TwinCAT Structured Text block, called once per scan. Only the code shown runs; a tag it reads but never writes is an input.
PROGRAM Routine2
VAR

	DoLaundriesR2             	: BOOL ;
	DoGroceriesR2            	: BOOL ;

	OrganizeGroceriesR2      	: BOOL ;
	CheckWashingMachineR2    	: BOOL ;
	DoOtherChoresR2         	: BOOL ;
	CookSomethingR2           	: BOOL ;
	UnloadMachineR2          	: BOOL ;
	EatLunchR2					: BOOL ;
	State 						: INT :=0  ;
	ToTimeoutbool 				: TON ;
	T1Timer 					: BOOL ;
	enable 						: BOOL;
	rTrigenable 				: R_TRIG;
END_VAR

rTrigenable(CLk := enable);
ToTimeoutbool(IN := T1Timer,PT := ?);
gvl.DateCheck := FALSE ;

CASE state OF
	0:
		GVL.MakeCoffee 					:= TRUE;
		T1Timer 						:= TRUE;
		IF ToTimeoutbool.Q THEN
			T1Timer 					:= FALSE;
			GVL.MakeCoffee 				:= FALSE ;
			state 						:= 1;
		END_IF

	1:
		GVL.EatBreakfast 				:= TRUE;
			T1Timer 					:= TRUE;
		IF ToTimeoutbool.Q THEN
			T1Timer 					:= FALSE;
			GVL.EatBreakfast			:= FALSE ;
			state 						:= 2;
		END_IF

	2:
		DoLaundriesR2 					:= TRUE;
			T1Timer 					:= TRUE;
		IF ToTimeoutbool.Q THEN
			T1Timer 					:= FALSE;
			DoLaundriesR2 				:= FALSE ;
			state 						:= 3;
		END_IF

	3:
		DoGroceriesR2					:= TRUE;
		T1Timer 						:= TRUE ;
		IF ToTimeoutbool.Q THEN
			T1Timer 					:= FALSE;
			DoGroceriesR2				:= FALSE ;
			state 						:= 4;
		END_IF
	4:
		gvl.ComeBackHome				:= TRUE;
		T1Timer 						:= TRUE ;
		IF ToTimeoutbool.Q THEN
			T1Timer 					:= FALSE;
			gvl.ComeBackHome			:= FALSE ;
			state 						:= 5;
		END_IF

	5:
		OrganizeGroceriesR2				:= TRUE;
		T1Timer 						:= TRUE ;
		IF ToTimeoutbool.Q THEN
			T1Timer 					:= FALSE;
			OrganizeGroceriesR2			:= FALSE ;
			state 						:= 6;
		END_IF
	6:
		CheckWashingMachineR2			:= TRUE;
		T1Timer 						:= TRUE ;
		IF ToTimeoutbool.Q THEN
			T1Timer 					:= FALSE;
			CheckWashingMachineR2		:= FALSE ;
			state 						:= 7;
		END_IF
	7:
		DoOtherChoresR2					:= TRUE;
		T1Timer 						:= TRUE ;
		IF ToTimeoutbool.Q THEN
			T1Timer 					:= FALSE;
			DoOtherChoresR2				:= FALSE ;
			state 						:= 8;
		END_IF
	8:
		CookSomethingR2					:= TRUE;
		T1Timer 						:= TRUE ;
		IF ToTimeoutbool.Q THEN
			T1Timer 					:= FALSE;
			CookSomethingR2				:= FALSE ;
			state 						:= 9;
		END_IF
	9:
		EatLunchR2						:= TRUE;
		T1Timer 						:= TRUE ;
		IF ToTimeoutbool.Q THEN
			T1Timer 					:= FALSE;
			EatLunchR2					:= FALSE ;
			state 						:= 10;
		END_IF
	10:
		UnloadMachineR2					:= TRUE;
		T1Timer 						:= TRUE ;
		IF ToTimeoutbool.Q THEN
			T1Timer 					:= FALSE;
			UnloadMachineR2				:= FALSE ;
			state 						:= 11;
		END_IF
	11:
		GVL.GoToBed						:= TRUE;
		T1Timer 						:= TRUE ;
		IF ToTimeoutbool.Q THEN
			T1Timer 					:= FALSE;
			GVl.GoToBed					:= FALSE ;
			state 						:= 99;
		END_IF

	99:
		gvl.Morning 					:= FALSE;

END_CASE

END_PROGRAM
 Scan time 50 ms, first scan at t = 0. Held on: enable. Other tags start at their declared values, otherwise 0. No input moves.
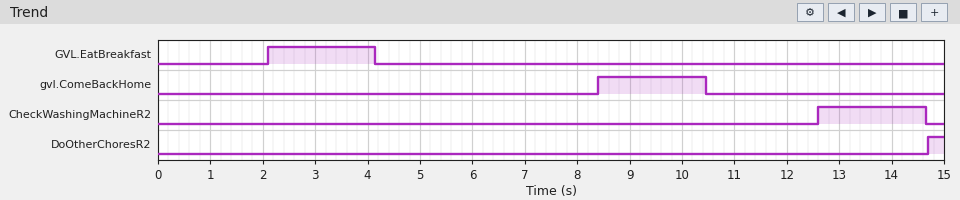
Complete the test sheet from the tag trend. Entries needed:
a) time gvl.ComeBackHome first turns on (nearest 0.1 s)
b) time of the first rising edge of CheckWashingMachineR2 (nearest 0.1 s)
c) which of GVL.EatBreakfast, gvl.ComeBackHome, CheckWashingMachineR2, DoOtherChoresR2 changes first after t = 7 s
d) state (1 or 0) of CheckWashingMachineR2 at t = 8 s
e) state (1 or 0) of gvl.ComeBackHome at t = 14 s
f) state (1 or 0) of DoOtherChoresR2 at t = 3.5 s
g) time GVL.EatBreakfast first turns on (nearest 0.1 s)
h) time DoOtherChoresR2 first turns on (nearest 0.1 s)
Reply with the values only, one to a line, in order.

8.4 s
12.6 s
gvl.ComeBackHome
0
0
0
2.1 s
14.7 s
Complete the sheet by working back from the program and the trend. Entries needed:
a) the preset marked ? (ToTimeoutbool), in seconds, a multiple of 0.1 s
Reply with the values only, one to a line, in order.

2.0 s
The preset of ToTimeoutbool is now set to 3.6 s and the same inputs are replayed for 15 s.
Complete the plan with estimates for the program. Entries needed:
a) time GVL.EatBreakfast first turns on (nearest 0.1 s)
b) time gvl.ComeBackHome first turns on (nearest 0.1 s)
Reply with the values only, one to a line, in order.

3.7 s
14.8 s
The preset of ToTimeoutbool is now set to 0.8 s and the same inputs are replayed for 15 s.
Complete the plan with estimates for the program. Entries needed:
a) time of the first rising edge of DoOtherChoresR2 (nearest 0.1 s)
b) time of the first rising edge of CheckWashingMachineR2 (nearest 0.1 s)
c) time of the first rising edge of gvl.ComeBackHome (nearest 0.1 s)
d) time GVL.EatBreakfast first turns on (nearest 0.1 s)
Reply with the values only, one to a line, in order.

6.3 s
5.4 s
3.6 s
0.9 s
